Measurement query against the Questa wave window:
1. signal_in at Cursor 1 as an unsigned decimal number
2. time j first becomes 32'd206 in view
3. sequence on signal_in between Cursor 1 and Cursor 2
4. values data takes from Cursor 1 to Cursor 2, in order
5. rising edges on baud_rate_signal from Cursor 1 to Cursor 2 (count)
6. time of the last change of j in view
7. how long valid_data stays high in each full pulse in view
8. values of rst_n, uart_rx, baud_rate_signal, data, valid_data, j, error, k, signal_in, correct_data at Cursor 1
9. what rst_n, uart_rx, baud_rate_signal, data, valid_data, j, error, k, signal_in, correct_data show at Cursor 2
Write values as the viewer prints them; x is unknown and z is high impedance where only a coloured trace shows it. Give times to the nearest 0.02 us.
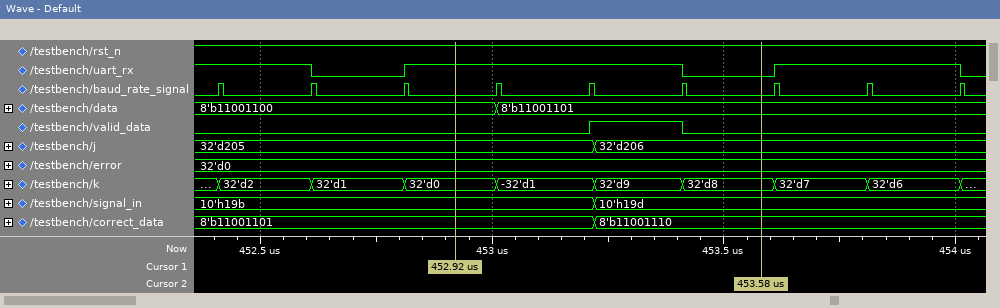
411
453.22 us
10'h19b, 10'h19d
8'b11001100, 8'b11001101
3
453.22 us
0.2 us
rst_n=1, uart_rx=1, baud_rate_signal=0, data=8'b11001100, valid_data=0, j=32'd205, error=32'd0, k=32'd0, signal_in=10'h19b, correct_data=8'b11001101
rst_n=1, uart_rx=0, baud_rate_signal=0, data=8'b11001101, valid_data=0, j=32'd206, error=32'd0, k=32'd8, signal_in=10'h19d, correct_data=8'b11001110
